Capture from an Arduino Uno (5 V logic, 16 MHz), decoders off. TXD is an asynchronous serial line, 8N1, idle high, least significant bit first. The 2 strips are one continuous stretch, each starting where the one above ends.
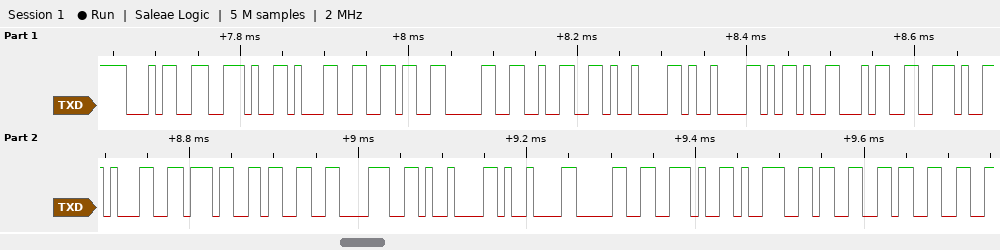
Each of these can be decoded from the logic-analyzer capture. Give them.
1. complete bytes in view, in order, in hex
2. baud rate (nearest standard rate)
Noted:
34 2E 31 36 30 32 09 09 2D 34 2E 31 37 33 38 09 09 30 2E 39 33 33
115200 baud
